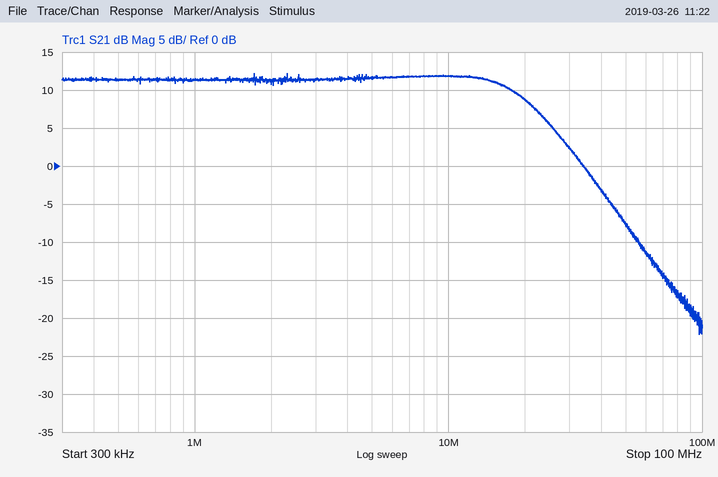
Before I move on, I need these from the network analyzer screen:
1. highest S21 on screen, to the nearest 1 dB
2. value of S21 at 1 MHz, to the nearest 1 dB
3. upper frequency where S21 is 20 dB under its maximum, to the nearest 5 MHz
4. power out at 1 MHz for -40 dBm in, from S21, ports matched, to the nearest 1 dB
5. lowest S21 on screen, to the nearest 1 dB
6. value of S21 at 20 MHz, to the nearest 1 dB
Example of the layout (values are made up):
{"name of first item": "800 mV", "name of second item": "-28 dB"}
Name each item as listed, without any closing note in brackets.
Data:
{"highest S21 on screen, to the nearest 1 dB": "12 dB", "value of S21 at 1 MHz, to the nearest 1 dB": "11 dB", "upper frequency where S21 is 20 dB under its maximum, to the nearest 5 MHz": "50 MHz", "power out at 1 MHz for -40 dBm in, from S21, ports matched, to the nearest 1 dB": "-29 dBm", "lowest S21 on screen, to the nearest 1 dB": "-22 dB", "value of S21 at 20 MHz, to the nearest 1 dB": "9 dB"}
